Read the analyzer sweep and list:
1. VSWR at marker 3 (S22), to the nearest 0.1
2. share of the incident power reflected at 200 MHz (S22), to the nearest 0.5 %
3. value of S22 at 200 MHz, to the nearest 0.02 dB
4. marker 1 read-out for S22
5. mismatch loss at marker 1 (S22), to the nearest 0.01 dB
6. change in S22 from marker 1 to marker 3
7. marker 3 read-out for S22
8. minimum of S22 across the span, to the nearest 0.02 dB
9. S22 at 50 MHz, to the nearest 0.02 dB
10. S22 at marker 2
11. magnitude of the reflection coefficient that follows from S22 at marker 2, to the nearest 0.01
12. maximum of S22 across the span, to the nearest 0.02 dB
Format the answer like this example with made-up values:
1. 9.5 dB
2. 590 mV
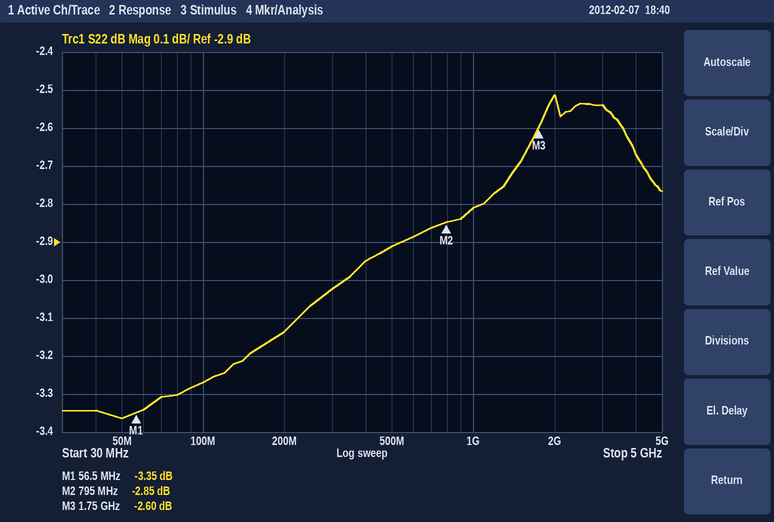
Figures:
1. 6.7
2. 48.5 %
3. -3.14 dB
4. -3.35 dB
5. 2.70 dB
6. 0.75 dB
7. -2.60 dB
8. -3.36 dB
9. -3.36 dB
10. -2.85 dB
11. 0.72
12. -2.52 dB
